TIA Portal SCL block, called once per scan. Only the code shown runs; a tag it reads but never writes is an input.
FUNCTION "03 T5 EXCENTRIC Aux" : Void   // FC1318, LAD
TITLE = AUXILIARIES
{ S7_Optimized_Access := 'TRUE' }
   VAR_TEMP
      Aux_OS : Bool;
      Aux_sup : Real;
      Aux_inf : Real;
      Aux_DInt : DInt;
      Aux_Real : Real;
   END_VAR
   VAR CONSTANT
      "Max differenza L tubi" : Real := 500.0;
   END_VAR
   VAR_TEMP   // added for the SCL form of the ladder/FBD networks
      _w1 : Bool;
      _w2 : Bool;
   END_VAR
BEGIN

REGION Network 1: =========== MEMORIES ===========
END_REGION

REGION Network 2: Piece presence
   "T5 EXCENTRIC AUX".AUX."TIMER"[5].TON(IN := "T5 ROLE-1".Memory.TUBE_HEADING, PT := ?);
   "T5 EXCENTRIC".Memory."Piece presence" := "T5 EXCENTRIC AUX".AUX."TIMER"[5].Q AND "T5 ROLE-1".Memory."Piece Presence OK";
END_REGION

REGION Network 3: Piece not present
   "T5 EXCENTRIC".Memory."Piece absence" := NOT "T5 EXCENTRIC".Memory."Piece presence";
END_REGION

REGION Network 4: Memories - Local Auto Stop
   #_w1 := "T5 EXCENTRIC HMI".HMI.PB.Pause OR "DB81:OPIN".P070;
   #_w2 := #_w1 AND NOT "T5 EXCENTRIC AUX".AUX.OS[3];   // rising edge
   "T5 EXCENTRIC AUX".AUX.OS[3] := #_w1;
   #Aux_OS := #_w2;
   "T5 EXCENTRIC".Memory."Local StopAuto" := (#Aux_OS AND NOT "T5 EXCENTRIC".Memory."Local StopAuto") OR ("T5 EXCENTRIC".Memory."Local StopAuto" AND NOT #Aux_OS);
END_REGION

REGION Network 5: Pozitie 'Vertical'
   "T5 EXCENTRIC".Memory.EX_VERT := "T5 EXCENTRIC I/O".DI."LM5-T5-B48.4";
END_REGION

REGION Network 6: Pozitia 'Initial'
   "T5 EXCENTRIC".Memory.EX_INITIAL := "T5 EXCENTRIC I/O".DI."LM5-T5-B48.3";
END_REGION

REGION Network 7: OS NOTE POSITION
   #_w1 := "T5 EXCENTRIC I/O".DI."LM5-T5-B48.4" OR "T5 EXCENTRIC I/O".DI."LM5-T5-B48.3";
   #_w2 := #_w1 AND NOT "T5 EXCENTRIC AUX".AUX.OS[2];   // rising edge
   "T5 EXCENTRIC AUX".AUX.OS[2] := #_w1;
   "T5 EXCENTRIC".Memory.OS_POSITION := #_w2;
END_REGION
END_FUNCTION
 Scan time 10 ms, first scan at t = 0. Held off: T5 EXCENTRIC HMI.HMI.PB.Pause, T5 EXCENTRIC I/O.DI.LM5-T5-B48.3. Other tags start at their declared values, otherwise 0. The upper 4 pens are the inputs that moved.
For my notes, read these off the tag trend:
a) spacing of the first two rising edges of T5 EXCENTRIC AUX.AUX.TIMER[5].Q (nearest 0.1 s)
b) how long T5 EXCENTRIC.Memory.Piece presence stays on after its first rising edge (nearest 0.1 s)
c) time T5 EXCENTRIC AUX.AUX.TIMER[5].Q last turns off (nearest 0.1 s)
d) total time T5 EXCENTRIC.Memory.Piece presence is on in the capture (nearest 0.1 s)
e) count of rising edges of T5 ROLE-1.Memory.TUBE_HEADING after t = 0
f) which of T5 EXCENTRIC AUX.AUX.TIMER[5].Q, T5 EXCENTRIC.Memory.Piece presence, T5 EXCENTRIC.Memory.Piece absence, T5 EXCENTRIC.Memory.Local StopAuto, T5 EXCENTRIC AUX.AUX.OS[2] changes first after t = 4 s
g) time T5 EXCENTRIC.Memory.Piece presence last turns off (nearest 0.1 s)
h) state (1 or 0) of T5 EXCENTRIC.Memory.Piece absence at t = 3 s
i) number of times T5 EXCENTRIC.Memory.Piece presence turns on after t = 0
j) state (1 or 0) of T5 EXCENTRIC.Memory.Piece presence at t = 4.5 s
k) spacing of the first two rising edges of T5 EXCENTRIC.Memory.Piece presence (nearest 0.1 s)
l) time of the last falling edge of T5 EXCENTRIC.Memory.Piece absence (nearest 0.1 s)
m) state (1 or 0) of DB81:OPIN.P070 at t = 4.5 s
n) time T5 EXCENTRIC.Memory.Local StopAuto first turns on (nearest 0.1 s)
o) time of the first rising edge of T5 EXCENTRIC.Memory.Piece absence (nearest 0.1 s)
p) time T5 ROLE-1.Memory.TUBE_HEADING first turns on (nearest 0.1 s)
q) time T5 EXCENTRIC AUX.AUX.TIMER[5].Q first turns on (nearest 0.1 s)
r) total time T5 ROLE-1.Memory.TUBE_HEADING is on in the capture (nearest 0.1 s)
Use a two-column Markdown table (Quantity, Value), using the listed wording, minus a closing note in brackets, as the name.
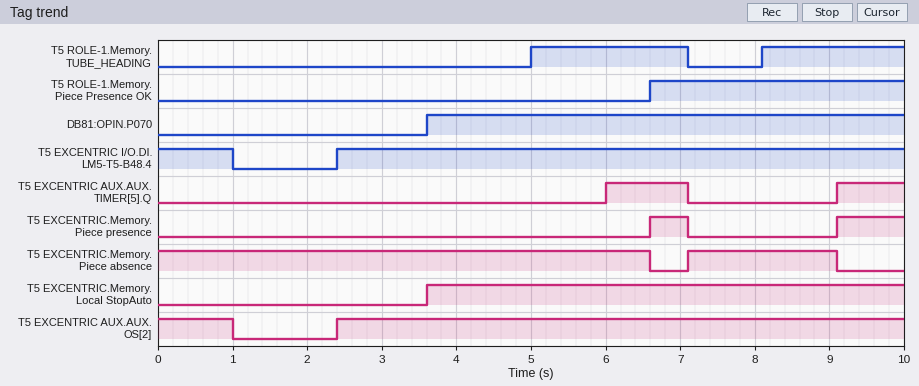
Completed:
| Quantity | Value |
|---|---|
| spacing of the first two rising edges of T5 EXCENTRIC AUX.AUX.TIMER[5].Q | 3.1 s |
| how long T5 EXCENTRIC.Memory.Piece presence stays on after its first rising edge | 0.5 s |
| time T5 EXCENTRIC AUX.AUX.TIMER[5].Q last turns off | 7.1 s |
| total time T5 EXCENTRIC.Memory.Piece presence is on in the capture | 1.4 s |
| count of rising edges of T5 ROLE-1.Memory.TUBE_HEADING after t = 0 | 2 |
| which of T5 EXCENTRIC AUX.AUX.TIMER[5].Q, T5 EXCENTRIC.Memory.Piece presence, T5 EXCENTRIC.Memory.Piece absence, T5 EXCENTRIC.Memory.Local StopAuto, T5 EXCENTRIC AUX.AUX.OS[2] changes first after t = 4 s | T5 EXCENTRIC AUX.AUX.TIMER[5].Q |
| time T5 EXCENTRIC.Memory.Piece presence last turns off | 7.1 s |
| state (1 or 0) of T5 EXCENTRIC.Memory.Piece absence at t = 3 s | 1 |
| number of times T5 EXCENTRIC.Memory.Piece presence turns on after t = 0 | 2 |
| state (1 or 0) of T5 EXCENTRIC.Memory.Piece presence at t = 4.5 s | 0 |
| spacing of the first two rising edges of T5 EXCENTRIC.Memory.Piece presence | 2.5 s |
| time of the last falling edge of T5 EXCENTRIC.Memory.Piece absence | 9.1 s |
| state (1 or 0) of DB81:OPIN.P070 at t = 4.5 s | 1 |
| time T5 EXCENTRIC.Memory.Local StopAuto first turns on | 3.6 s |
| time of the first rising edge of T5 EXCENTRIC.Memory.Piece absence | 7.1 s |
| time T5 ROLE-1.Memory.TUBE_HEADING first turns on | 5.0 s |
| time T5 EXCENTRIC AUX.AUX.TIMER[5].Q first turns on | 6.0 s |
| total time T5 ROLE-1.Memory.TUBE_HEADING is on in the capture | 4.0 s |
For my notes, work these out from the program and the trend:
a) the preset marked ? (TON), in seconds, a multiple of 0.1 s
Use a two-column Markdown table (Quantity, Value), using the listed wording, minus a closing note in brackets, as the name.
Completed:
| Quantity | Value |
|---|---|
| the preset marked ? (TON), in seconds, a multiple of 0.1 s | 1.0 s |
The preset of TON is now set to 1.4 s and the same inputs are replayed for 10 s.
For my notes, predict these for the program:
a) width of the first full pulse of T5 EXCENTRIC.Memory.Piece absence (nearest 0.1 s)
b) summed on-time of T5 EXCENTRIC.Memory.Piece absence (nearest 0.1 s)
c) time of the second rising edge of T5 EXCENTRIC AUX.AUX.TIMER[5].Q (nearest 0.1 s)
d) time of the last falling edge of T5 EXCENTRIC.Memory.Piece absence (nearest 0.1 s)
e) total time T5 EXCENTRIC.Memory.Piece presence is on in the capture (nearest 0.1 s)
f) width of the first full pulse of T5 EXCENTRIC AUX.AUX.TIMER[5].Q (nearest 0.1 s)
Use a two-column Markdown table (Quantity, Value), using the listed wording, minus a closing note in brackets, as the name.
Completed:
| Quantity | Value |
|---|---|
| width of the first full pulse of T5 EXCENTRIC.Memory.Piece absence | 2.4 s |
| summed on-time of T5 EXCENTRIC.Memory.Piece absence | 9.0 s |
| time of the second rising edge of T5 EXCENTRIC AUX.AUX.TIMER[5].Q | 9.5 s |
| time of the last falling edge of T5 EXCENTRIC.Memory.Piece absence | 9.5 s |
| total time T5 EXCENTRIC.Memory.Piece presence is on in the capture | 1.0 s |
| width of the first full pulse of T5 EXCENTRIC AUX.AUX.TIMER[5].Q | 0.7 s |
